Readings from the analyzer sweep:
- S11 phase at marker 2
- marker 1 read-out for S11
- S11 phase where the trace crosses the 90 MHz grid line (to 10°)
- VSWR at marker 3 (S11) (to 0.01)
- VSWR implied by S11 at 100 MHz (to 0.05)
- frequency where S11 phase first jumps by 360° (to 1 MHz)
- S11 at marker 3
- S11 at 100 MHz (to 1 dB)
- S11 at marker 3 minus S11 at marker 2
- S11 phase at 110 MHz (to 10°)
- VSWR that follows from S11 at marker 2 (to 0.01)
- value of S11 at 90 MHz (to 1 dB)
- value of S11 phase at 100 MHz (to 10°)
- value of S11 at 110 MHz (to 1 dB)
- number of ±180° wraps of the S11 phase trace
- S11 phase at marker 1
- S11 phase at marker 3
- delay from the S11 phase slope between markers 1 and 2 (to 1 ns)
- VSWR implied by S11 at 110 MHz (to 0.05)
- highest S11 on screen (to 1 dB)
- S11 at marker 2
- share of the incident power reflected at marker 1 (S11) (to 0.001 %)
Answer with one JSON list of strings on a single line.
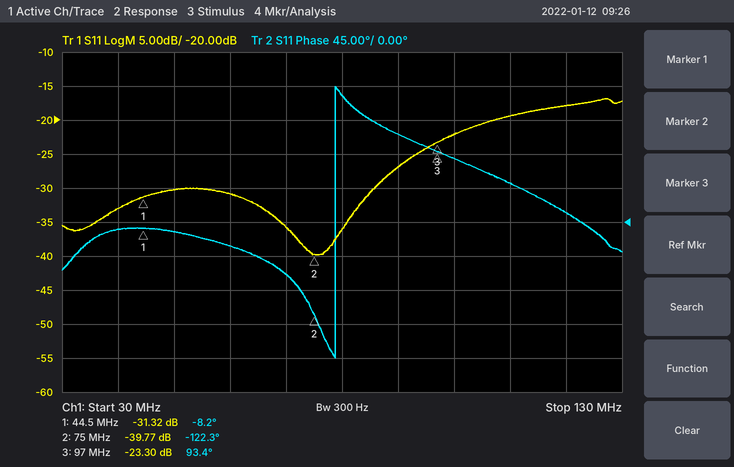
["-122.3°", "-31.32 dB", "120°", "1.15", "1.15", "79 MHz", "-23.30 dB", "-22 dB", "16.47 dB", "50°", "1.02", "-27 dB", "80°", "-19 dB", "1", "-8.2°", "93.4°", "10 ns", "1.25", "-17 dB", "-39.77 dB", "0.074 %"]
